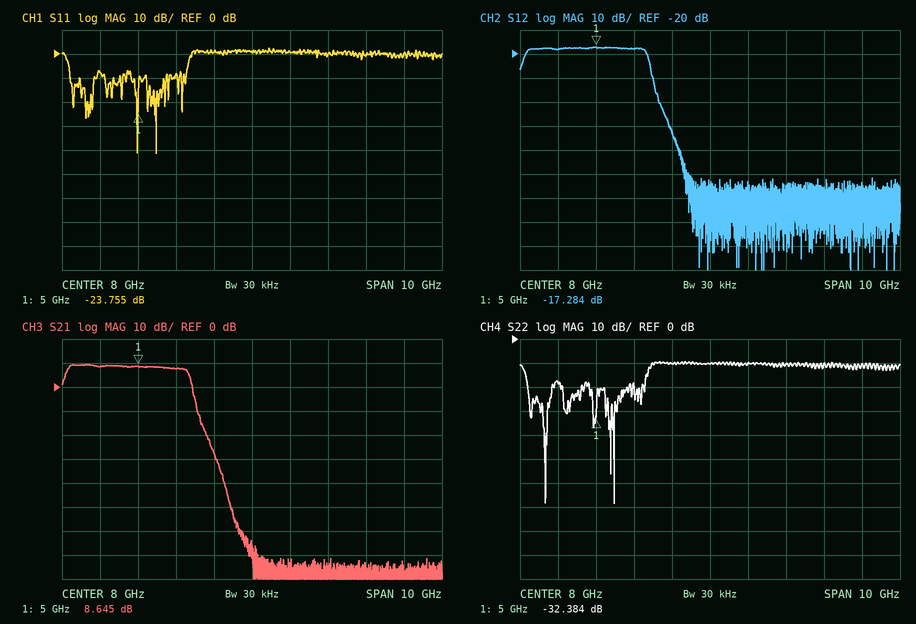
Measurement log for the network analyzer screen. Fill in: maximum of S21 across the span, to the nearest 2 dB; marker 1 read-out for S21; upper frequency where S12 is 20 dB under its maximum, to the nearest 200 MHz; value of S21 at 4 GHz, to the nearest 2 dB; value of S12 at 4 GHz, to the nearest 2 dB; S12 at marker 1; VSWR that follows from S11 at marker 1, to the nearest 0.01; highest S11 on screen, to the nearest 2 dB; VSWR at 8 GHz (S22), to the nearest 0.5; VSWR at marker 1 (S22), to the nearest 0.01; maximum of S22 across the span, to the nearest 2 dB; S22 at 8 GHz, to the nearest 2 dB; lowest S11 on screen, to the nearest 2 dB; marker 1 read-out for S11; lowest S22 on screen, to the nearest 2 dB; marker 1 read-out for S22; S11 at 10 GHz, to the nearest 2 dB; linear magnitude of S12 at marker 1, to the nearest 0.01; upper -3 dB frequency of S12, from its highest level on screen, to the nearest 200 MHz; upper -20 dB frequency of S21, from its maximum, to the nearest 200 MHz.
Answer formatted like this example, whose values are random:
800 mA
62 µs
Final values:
10 dB
8.645 dB
6.6 GHz
8 dB
-18 dB
-17.284 dB
1.14
2 dB
2.0
1.05
-10 dB
-10 dB
-42 dB
-23.755 dB
-68 dB
-32.384 dB
0 dB
0.14
6.4 GHz
6.6 GHz
